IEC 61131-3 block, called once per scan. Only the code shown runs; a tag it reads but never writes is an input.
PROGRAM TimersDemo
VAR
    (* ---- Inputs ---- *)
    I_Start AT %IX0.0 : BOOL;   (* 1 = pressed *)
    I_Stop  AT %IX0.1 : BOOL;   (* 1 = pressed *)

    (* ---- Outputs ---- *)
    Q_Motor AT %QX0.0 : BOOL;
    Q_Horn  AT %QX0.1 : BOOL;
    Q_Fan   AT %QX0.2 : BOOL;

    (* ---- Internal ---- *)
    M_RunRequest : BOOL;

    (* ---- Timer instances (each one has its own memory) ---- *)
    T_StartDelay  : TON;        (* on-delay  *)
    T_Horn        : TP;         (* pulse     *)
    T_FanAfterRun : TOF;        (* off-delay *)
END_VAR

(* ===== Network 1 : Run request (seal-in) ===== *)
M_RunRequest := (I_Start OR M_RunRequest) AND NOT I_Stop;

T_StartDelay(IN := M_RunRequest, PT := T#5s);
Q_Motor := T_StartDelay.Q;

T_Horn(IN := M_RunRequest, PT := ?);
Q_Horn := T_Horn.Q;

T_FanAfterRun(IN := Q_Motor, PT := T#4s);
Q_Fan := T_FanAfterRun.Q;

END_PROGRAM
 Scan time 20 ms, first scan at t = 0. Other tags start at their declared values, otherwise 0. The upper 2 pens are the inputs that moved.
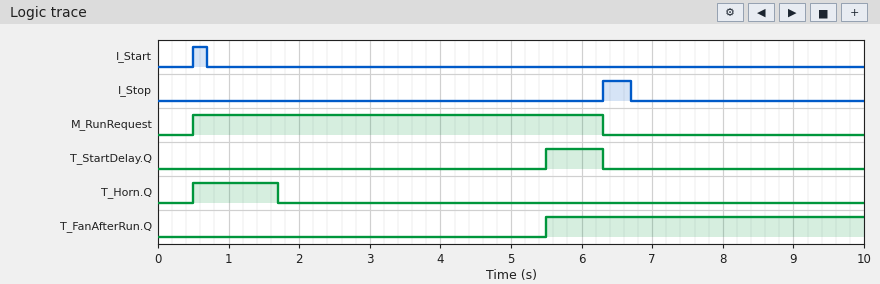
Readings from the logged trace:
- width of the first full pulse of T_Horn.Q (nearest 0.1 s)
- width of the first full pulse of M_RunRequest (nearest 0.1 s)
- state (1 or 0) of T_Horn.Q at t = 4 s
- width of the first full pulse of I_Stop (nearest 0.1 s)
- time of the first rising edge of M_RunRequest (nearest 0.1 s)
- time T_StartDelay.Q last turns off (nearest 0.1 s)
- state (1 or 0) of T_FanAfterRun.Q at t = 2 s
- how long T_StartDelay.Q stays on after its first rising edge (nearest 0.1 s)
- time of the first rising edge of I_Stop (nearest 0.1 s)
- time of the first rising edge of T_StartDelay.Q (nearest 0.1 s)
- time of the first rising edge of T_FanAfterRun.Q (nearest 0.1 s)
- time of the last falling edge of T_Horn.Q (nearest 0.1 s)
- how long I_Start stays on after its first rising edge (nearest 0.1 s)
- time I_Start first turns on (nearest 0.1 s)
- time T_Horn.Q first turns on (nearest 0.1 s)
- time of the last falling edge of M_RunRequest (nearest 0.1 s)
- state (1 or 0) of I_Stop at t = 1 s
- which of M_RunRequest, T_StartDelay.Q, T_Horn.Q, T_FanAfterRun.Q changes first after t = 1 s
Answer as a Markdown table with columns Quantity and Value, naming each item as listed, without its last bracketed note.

| Quantity | Value |
|---|---|
| width of the first full pulse of T_Horn.Q | 1.2 s |
| width of the first full pulse of M_RunRequest | 5.8 s |
| state (1 or 0) of T_Horn.Q at t = 4 s | 0 |
| width of the first full pulse of I_Stop | 0.4 s |
| time of the first rising edge of M_RunRequest | 0.5 s |
| time T_StartDelay.Q last turns off | 6.3 s |
| state (1 or 0) of T_FanAfterRun.Q at t = 2 s | 0 |
| how long T_StartDelay.Q stays on after its first rising edge | 0.8 s |
| time of the first rising edge of I_Stop | 6.3 s |
| time of the first rising edge of T_StartDelay.Q | 5.5 s |
| time of the first rising edge of T_FanAfterRun.Q | 5.5 s |
| time of the last falling edge of T_Horn.Q | 1.7 s |
| how long I_Start stays on after its first rising edge | 0.2 s |
| time I_Start first turns on | 0.5 s |
| time T_Horn.Q first turns on | 0.5 s |
| time of the last falling edge of M_RunRequest | 6.3 s |
| state (1 or 0) of I_Stop at t = 1 s | 0 |
| which of M_RunRequest, T_StartDelay.Q, T_Horn.Q, T_FanAfterRun.Q changes first after t = 1 s | T_Horn.Q |
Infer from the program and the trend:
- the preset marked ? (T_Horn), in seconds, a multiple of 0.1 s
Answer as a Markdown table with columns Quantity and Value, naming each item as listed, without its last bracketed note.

| Quantity | Value |
|---|---|
| the preset marked ? (T_Horn), in seconds, a multiple of 0.1 s | 1.2 s |
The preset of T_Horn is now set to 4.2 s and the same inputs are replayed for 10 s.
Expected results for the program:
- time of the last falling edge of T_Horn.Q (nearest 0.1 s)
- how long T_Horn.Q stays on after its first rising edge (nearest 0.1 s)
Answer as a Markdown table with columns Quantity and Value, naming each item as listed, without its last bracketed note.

| Quantity | Value |
|---|---|
| time of the last falling edge of T_Horn.Q | 4.7 s |
| how long T_Horn.Q stays on after its first rising edge | 4.2 s |
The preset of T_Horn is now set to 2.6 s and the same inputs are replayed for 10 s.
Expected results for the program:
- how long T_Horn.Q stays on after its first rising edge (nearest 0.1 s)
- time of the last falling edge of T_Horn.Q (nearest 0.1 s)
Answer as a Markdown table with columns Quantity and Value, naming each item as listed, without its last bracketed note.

| Quantity | Value |
|---|---|
| how long T_Horn.Q stays on after its first rising edge | 2.6 s |
| time of the last falling edge of T_Horn.Q | 3.1 s |
